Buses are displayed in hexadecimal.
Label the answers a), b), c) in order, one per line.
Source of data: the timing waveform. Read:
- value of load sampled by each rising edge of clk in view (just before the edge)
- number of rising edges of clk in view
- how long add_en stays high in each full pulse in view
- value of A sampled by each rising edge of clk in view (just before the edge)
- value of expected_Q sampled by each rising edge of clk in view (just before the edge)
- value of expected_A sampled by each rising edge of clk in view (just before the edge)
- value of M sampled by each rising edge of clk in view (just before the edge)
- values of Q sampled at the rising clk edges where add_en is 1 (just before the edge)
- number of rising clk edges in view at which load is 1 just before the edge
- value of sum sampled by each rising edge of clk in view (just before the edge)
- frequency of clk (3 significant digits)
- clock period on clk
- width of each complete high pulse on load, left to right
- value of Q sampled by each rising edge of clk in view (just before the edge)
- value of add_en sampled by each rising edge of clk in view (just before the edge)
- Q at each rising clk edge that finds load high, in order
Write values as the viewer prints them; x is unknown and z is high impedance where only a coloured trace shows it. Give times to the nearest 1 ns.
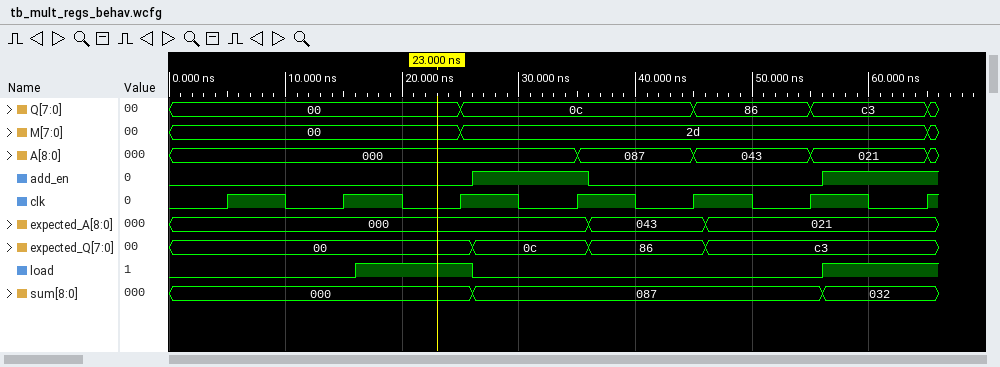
a) 0 0 1 0 0 0 1
b) 7
c) 10 ns
d) 000, 000, 000, 000, 087, 043, 021
e) 00, 00, 00, 0c, 86, c3, c3
f) 000, 000, 000, 000, 043, 021, 021
g) 00, 00, 00, 2d, 2d, 2d, 2d
h) 0c, c3
i) 2
j) 000, 000, 000, 087, 087, 087, 032
k) 100 MHz
l) 10 ns
m) 10 ns
n) 00, 00, 00, 0c, 0c, 86, c3
o) 0 0 0 1 0 0 1
p) 00, c3
